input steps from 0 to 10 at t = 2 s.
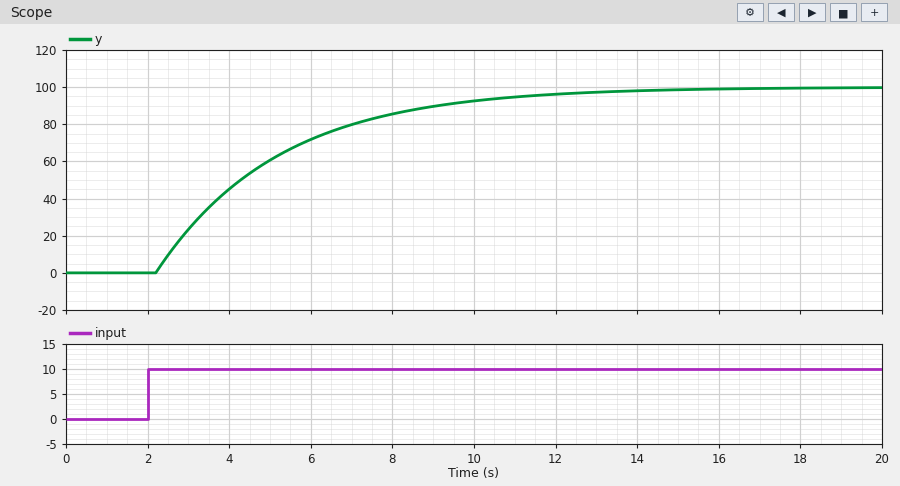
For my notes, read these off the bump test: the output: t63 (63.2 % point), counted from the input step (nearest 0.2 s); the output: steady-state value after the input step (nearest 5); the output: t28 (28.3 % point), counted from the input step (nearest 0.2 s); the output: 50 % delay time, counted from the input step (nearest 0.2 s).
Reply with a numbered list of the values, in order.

1. 3.2 s
2. 100
3. 1.2 s
4. 2.2 s
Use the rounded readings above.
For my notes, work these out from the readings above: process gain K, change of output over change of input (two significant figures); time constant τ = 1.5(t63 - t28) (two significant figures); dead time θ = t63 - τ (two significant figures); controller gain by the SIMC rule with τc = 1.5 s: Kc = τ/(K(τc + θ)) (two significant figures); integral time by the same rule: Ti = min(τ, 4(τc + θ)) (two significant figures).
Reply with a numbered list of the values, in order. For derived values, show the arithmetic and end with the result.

1. (100 - 0) / 10 = 10
2. 1.5 × (3.2 - 1.2) = 3.0 s
3. 3.2 - 3 = 0.20 s
4. 3 / (10 × (1.5 + 0.2)) = 0.18
5. min(3, 4 × (1.5 + 0.2)) = 3.0 s
